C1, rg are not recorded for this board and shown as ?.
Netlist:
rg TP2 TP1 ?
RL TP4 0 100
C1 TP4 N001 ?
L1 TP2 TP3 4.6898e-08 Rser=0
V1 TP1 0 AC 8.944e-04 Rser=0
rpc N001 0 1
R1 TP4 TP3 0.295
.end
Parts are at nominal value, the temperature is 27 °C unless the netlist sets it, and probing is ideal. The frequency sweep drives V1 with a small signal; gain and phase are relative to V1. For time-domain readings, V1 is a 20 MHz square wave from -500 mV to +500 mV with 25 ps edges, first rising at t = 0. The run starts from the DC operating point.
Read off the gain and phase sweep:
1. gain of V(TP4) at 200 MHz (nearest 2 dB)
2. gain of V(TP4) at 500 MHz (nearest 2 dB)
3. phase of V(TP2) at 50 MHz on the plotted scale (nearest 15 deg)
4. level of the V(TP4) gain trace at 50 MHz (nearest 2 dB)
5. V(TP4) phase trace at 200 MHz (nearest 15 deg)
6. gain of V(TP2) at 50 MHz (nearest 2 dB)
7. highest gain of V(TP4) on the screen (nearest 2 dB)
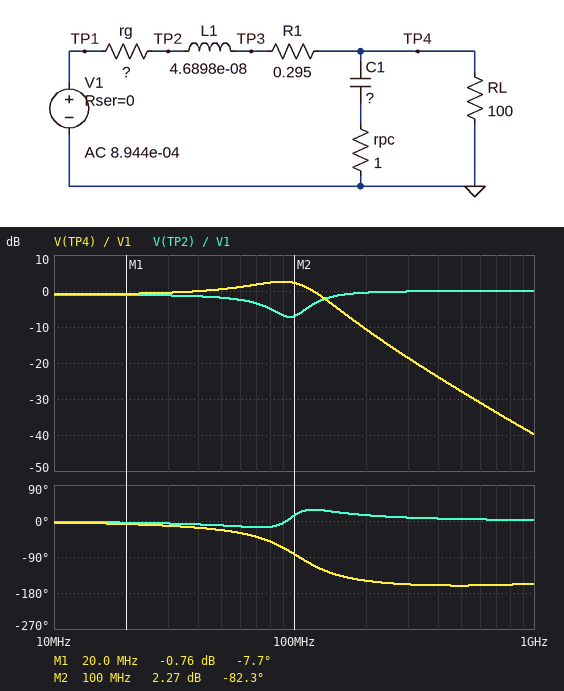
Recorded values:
-10 dB
-28 dB
-15 deg
0 dB
-150 deg
-2 dB
2 dB
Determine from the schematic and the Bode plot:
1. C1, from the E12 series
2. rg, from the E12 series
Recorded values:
56 pF
12 Ω
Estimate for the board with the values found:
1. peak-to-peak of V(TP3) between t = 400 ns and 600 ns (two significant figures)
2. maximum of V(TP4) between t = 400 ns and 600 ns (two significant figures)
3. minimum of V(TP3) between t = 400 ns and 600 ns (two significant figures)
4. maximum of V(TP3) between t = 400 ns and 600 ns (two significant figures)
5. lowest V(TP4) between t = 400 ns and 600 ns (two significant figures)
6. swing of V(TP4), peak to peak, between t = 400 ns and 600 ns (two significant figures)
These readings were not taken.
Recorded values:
1.4 V
720 mV
-720 mV
720 mV
-720 mV
1.4 V
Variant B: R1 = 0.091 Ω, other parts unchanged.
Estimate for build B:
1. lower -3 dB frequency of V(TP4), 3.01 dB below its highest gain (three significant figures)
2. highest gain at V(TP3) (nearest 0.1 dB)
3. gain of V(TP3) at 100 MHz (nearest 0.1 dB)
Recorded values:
32.4 MHz
2.7 dB
2.4 dB
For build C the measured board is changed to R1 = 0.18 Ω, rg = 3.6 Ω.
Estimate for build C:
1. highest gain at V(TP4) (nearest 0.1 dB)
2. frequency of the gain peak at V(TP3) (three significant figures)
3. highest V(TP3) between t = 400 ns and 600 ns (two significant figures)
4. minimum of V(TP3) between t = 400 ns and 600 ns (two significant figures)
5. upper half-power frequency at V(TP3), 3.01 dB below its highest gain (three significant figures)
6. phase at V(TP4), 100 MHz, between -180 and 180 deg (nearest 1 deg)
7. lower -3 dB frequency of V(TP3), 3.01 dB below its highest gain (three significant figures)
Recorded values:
6.9 dB
94.5 MHz
970 mV
-970 mV
115 MHz
-89 deg
68.0 MHz
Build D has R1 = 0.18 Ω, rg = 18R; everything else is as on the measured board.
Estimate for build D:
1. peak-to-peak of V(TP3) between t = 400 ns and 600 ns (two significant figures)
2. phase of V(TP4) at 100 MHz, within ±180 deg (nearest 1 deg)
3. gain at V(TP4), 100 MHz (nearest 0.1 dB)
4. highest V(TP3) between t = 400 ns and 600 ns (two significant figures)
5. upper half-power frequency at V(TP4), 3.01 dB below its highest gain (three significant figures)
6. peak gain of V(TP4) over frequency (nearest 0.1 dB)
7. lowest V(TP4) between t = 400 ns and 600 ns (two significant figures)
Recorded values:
1.2 V
-80 deg
0.1 dB
610 mV
126 MHz
0.6 dB
-610 mV
